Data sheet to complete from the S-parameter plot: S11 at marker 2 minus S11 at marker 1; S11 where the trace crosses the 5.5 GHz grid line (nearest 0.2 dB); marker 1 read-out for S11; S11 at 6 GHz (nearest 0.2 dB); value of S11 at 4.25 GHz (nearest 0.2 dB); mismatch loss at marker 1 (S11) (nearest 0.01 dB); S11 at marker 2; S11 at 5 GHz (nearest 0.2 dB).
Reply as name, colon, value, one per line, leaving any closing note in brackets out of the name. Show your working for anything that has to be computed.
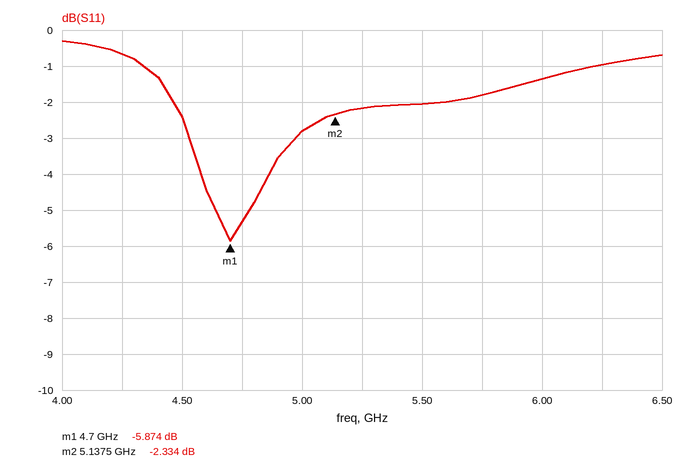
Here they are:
S11 at marker 2 minus S11 at marker 1: -2.334 − (-5.874) = 3.540 dB
S11 where the trace crosses the 5.5 GHz grid line: -2.0 dB
marker 1 read-out for S11: -5.874 dB
S11 at 6 GHz: -1.4 dB
value of S11 at 4.25 GHz: -0.6 dB
mismatch loss at marker 1 (S11): −10 log10(1 − 10^(-5.874/10)) ≈ 1.30 dB
S11 at marker 2: -2.334 dB
S11 at 5 GHz: -2.8 dB
